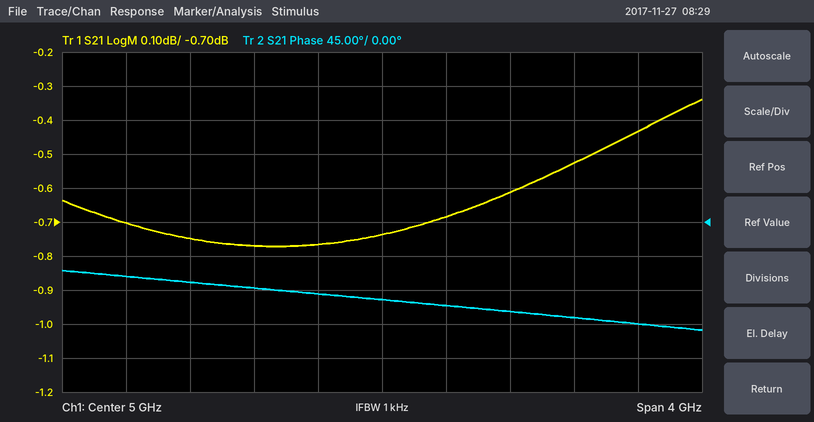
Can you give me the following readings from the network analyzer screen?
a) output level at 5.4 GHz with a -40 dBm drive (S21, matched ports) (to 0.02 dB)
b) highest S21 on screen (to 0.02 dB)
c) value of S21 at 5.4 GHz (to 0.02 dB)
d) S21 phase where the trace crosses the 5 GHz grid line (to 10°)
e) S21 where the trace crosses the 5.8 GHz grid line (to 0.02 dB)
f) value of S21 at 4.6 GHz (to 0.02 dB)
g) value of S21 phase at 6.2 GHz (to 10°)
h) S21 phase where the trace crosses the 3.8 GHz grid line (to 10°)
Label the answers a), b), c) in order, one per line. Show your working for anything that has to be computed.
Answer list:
a) -40 dBm + (-0.68 dB) = -40.68 dBm
b) -0.34 dB
c) -0.68 dB
d) -100°
e) -0.62 dB
f) -0.76 dB
g) -130°
h) -80°
